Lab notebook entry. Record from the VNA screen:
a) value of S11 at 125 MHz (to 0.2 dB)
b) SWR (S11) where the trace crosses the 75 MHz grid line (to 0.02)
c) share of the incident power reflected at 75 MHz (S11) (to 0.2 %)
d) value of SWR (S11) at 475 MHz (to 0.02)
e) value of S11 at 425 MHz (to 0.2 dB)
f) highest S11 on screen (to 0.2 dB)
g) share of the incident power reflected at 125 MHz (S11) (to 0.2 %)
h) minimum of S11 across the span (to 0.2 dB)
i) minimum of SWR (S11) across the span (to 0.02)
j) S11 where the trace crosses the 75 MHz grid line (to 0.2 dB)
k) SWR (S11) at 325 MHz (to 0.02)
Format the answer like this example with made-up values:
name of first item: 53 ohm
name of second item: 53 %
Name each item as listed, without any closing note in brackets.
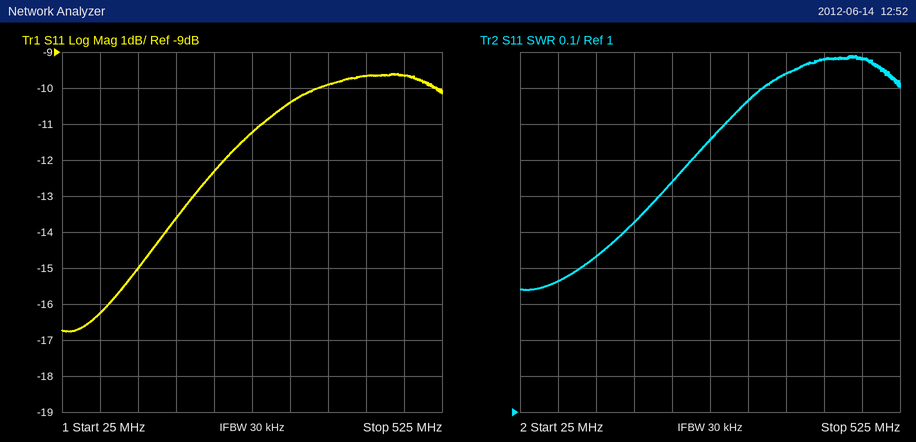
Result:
value of S11 at 125 MHz: -15.0 dB
SWR (S11) where the trace crosses the 75 MHz grid line: 1.36
share of the incident power reflected at 75 MHz (S11): 2.4 %
value of SWR (S11) at 475 MHz: 1.98
value of S11 at 425 MHz: -9.6 dB
highest S11 on screen: -9.6 dB
share of the incident power reflected at 125 MHz (S11): 3.2 %
minimum of S11 across the span: -16.8 dB
minimum of SWR (S11) across the span: 1.34
S11 where the trace crosses the 75 MHz grid line: -16.2 dB
SWR (S11) at 325 MHz: 1.86
